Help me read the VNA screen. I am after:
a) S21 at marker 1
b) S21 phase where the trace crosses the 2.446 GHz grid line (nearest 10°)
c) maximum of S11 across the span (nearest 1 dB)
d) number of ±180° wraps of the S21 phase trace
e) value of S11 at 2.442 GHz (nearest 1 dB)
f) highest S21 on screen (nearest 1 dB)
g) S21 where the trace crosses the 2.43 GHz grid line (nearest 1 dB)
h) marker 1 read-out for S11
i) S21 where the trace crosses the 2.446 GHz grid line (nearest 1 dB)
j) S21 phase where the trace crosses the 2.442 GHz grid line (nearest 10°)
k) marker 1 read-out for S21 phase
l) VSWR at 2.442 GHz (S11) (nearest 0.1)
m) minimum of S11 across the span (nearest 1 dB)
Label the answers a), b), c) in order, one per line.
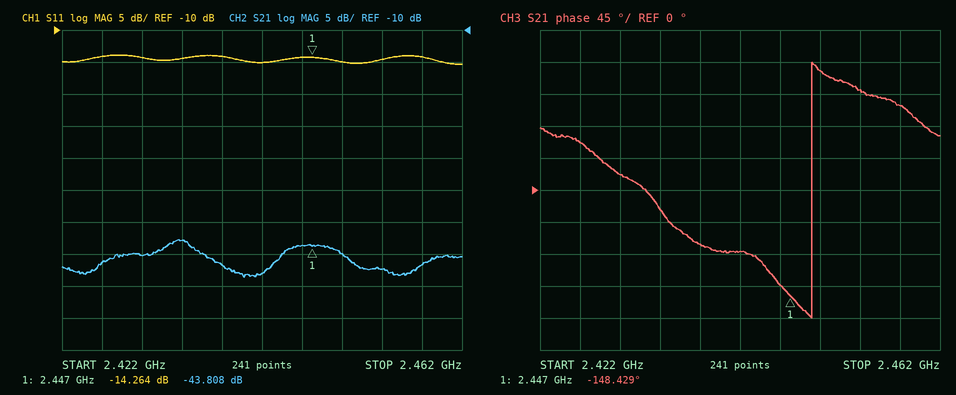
a) -43.808 dB
b) -130°
c) -14 dB
d) 1
e) -15 dB
f) -43 dB
g) -45 dB
h) -14.264 dB
i) -44 dB
j) -90°
k) -148.429°
l) 1.4
m) -15 dB
